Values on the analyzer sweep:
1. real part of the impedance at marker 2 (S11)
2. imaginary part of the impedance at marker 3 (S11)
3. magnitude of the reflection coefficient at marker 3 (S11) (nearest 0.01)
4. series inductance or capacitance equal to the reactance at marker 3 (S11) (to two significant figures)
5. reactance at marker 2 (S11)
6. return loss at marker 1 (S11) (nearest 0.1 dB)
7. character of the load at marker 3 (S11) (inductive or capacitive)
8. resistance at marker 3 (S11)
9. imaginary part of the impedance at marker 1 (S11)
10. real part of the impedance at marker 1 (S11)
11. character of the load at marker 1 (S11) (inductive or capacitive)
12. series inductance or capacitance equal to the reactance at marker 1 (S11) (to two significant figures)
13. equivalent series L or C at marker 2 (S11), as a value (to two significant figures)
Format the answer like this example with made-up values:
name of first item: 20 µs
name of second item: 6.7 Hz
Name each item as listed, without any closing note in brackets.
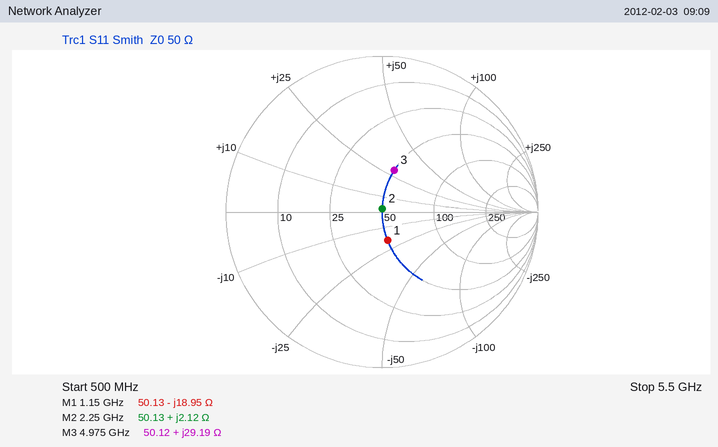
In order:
real part of the impedance at marker 2: 50.13 Ω
imaginary part of the impedance at marker 3: +29.19 Ω
magnitude of the reflection coefficient at marker 3 (S11): 0.28
series inductance or capacitance equal to the reactance at marker 3 (S11): 930 pH
reactance at marker 2: +2.12 Ω
return loss at marker 1 (S11): 14.6 dB
character of the load at marker 3 (S11): inductive
resistance at marker 3: 50.12 Ω
imaginary part of the impedance at marker 1: -18.95 Ω
real part of the impedance at marker 1: 50.13 Ω
character of the load at marker 1 (S11): capacitive
series inductance or capacitance equal to the reactance at marker 1 (S11): 7.3 pF
equivalent series L or C at marker 2 (S11), as a value: 150 pH
